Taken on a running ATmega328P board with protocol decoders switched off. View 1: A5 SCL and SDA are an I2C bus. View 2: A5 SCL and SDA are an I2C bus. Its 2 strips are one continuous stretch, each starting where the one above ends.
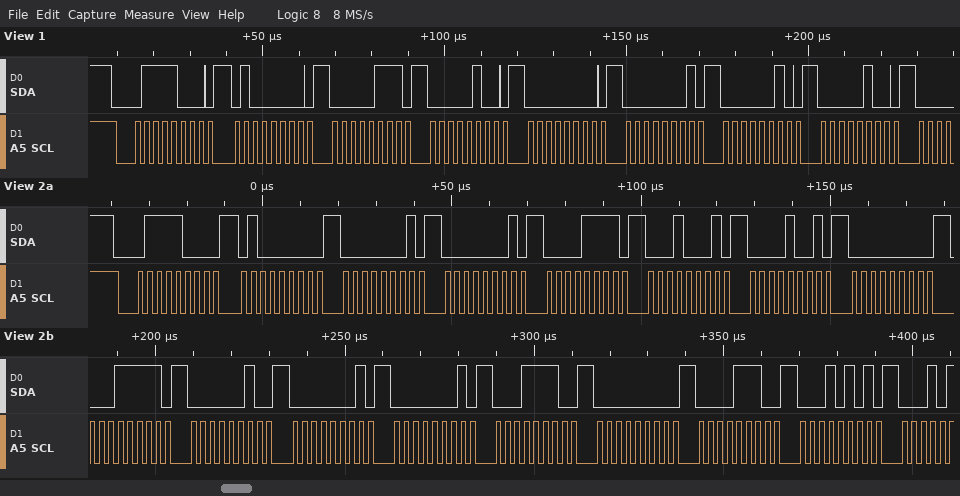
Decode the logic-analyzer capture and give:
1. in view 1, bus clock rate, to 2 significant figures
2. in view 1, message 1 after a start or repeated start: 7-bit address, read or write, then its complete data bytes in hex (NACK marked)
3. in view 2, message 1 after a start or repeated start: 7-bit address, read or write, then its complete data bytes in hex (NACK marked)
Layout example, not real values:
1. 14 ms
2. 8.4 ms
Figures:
1. 400 kHz
2. 0x3C write: 40 07 04 00 01 02 04
3. 0x3C write: 40 01 01 0F 11 09 00 1F 02 01 01 1E 00 0E 15
